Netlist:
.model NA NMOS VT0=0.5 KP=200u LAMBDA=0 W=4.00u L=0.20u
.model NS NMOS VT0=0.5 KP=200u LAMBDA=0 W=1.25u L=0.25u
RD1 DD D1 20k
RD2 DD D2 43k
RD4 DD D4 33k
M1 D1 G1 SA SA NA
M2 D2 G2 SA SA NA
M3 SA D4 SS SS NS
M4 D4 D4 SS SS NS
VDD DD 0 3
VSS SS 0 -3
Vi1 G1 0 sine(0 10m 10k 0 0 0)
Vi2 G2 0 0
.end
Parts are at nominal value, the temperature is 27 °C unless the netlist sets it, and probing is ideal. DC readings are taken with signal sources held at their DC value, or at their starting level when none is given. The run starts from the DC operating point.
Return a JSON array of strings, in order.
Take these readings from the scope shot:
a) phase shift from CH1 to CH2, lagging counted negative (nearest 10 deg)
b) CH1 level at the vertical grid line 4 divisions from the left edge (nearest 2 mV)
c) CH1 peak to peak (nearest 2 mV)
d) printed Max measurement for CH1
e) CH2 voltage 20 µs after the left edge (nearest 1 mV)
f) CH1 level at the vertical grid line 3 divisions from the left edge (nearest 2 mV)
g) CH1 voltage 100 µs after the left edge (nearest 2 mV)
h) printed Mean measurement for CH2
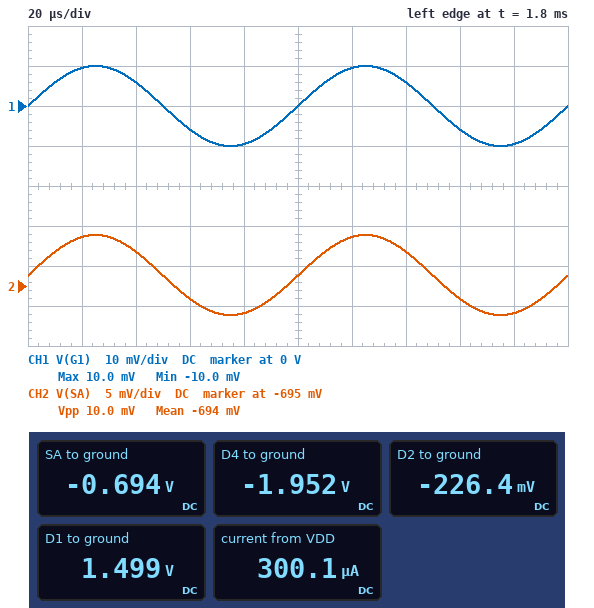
["0 deg", "-10 mV", "20 mV", "10.0 mV", "-689 mV", "-6 mV", "0 V", "-694 mV"]
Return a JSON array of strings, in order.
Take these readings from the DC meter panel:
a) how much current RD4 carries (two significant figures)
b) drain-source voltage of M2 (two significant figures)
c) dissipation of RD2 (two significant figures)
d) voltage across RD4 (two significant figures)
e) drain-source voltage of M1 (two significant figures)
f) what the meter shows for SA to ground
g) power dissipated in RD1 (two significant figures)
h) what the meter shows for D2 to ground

["150 µA", "470 mV", "240 µW", "5.0 V", "2.2 V", "-0.694 V", "110 µW", "-226.4 mV"]
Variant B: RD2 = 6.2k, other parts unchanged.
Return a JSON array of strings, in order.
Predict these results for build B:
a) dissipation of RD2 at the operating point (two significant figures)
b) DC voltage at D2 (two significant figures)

["35 µW", "2.5 V"]
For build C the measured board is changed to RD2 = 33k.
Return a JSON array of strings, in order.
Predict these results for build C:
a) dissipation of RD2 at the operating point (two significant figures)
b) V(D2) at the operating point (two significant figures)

["190 µW", "520 mV"]
